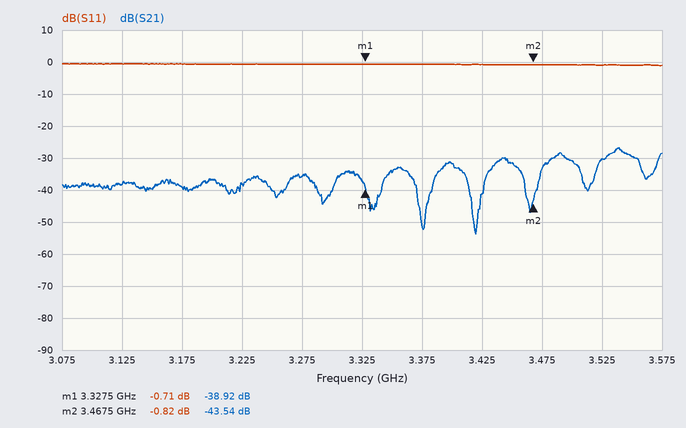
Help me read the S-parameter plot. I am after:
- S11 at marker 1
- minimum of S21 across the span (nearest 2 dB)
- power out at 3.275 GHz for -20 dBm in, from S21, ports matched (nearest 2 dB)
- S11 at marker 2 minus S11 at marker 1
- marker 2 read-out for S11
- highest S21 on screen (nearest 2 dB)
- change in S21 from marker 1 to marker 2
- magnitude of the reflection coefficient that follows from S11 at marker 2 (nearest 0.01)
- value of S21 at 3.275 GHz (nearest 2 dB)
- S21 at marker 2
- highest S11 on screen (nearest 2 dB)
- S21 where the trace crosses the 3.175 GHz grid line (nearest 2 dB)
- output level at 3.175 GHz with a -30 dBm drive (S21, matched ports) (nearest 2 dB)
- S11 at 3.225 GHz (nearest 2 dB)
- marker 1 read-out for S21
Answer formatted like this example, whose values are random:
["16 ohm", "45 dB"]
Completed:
["-0.71 dB", "-54 dB", "-56 dBm", "-0.11 dB", "-0.82 dB", "-26 dB", "-4.62 dB", "0.91", "-36 dB", "-43.54 dB", "0 dB", "-40 dB", "-70 dBm", "0 dB", "-38.92 dB"]
